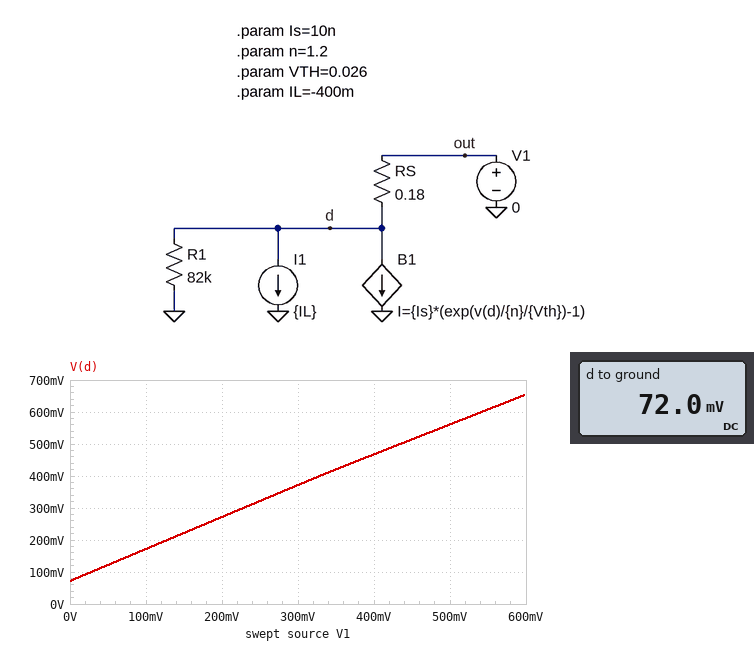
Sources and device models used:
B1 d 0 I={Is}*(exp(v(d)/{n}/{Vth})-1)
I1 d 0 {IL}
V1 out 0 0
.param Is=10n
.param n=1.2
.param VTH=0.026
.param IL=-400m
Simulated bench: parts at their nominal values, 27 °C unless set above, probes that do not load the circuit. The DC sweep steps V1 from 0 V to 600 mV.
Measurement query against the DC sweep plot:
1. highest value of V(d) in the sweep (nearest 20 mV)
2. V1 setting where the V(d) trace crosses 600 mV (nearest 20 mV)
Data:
660 mV
540 mV
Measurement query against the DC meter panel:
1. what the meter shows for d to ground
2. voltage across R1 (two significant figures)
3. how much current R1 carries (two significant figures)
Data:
72.0 mV
72 mV
880 nA
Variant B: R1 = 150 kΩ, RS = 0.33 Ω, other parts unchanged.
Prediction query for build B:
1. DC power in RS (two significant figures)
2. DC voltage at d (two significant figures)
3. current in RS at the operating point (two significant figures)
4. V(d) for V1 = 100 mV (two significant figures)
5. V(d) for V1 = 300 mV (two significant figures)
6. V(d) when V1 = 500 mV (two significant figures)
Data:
53 mW
130 mV
400 mA
230 mV
430 mV
610 mV
